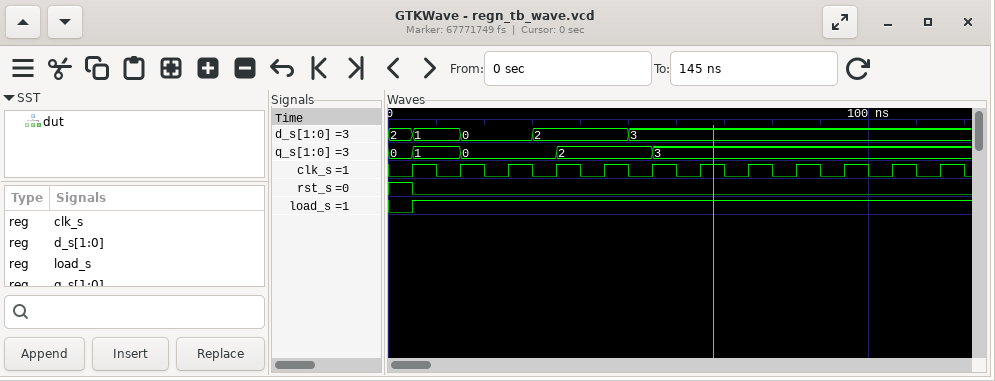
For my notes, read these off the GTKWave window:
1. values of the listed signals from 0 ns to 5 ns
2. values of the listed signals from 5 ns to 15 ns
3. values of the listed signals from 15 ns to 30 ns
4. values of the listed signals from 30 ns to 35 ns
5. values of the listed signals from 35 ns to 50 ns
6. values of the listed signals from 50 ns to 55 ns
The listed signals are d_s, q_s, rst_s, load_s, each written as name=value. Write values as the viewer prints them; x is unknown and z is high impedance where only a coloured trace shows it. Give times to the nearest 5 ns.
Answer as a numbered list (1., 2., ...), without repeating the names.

1. d_s=2, q_s=0, rst_s=1, load_s=0
2. d_s=1, q_s=1, rst_s=0, load_s=1
3. d_s=0, q_s=0, rst_s=0, load_s=1
4. d_s=2, q_s=0, rst_s=0, load_s=1
5. d_s=2, q_s=2, rst_s=0, load_s=1
6. d_s=3, q_s=2, rst_s=0, load_s=1
